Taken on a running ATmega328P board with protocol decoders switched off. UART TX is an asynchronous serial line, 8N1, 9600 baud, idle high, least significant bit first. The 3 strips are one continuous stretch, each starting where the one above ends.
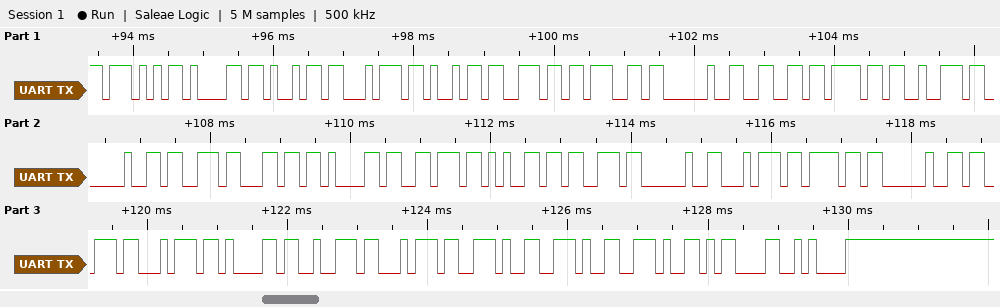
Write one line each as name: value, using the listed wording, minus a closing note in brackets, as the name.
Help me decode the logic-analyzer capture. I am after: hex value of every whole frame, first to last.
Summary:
hex value of every whole frame, first to last: 57 61 69 74 69 6E 67 20 66 6F 72 20 73 6C 61 76 65 73 20 74 6F 20 73 74 61 72 74 2E 2E 2E 0D 0A
